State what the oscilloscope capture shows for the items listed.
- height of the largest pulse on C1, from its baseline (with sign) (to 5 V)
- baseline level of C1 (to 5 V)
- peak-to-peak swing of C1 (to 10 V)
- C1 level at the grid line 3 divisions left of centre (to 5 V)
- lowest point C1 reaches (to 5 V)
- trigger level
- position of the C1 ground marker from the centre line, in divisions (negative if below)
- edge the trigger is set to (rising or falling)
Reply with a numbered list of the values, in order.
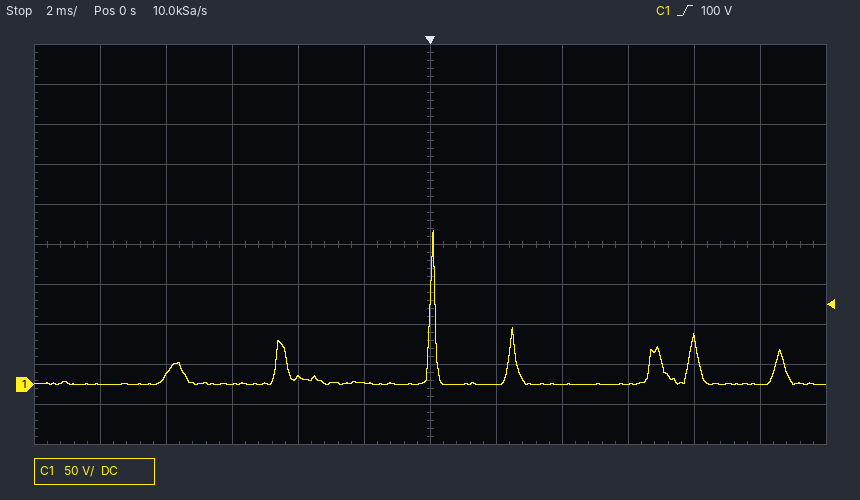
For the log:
1. +190 V
2. 0 V
3. 190 V
4. 0 V
5. 0 V
6. 100 V
7. -3.5 div
8. rising
